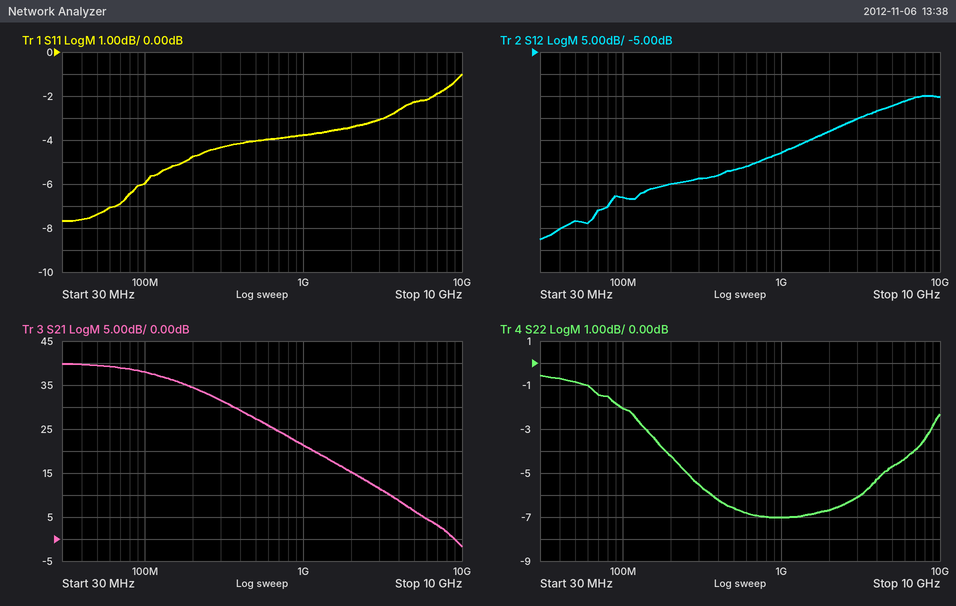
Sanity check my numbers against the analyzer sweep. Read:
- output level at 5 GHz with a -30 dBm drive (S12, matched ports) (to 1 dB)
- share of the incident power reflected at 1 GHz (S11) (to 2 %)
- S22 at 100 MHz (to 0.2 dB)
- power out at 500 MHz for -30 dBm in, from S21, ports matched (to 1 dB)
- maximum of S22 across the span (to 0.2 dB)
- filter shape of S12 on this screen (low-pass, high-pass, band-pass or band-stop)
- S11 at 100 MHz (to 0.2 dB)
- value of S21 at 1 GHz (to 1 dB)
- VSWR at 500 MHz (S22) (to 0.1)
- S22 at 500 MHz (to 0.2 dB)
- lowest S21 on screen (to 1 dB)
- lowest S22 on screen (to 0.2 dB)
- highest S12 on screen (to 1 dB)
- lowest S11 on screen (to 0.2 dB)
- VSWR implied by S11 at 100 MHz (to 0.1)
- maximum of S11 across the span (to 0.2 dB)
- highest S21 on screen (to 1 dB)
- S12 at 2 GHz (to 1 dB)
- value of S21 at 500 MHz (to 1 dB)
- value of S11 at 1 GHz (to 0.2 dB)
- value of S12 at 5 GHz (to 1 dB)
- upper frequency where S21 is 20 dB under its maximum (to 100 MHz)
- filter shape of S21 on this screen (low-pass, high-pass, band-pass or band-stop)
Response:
-47 dBm
42 %
-2.0 dB
-3 dBm
-0.6 dB
high-pass
-6.0 dB
21 dB
2.8
-6.6 dB
-2 dB
-7.0 dB
-15 dB
-7.6 dB
3.0
-1.0 dB
40 dB
-23 dB
27 dB
-3.8 dB
-17 dB
1.2 GHz
low-pass
